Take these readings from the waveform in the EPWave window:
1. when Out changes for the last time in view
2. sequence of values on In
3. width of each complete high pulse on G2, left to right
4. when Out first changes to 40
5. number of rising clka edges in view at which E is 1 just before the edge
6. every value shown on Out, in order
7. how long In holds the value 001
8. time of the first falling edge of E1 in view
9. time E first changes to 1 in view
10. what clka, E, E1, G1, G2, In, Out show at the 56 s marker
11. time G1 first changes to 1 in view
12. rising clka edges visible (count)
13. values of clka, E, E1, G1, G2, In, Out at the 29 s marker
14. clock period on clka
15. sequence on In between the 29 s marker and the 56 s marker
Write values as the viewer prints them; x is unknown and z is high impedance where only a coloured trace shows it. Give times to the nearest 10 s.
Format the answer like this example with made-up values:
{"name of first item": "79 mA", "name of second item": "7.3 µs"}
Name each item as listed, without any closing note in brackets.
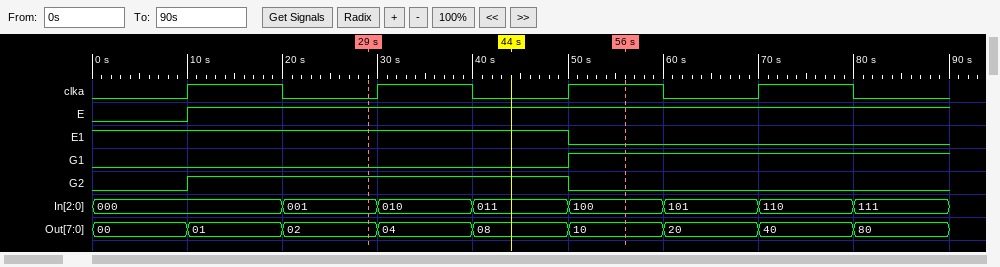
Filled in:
{"when Out changes for the last time in view": "80 s", "sequence of values on In": "000, 001, 010, 011, 100, 101, 110, 111", "width of each complete high pulse on G2, left to right": "40 s", "when Out first changes to 40": "70 s", "number of rising clka edges in view at which E is 1 just before the edge": "3", "every value shown on Out, in order": "00, 01, 02, 04, 08, 10, 20, 40, 80", "how long In holds the value 001": "10 s", "time of the first falling edge of E1 in view": "50 s", "time E first changes to 1 in view": "10 s", "what clka, E, E1, G1, G2, In, Out show at the 56 s marker": "clka=1, E=1, E1=0, G1=1, G2=0, In=100, Out=10", "time G1 first changes to 1 in view": "50 s", "rising clka edges visible": "4", "values of clka, E, E1, G1, G2, In, Out at the 29 s marker": "clka=0, E=1, E1=1, G1=0, G2=1, In=001, Out=02", "clock period on clka": "20 s", "sequence on In between the 29 s marker and the 56 s marker": "001, 010, 011, 100"}
